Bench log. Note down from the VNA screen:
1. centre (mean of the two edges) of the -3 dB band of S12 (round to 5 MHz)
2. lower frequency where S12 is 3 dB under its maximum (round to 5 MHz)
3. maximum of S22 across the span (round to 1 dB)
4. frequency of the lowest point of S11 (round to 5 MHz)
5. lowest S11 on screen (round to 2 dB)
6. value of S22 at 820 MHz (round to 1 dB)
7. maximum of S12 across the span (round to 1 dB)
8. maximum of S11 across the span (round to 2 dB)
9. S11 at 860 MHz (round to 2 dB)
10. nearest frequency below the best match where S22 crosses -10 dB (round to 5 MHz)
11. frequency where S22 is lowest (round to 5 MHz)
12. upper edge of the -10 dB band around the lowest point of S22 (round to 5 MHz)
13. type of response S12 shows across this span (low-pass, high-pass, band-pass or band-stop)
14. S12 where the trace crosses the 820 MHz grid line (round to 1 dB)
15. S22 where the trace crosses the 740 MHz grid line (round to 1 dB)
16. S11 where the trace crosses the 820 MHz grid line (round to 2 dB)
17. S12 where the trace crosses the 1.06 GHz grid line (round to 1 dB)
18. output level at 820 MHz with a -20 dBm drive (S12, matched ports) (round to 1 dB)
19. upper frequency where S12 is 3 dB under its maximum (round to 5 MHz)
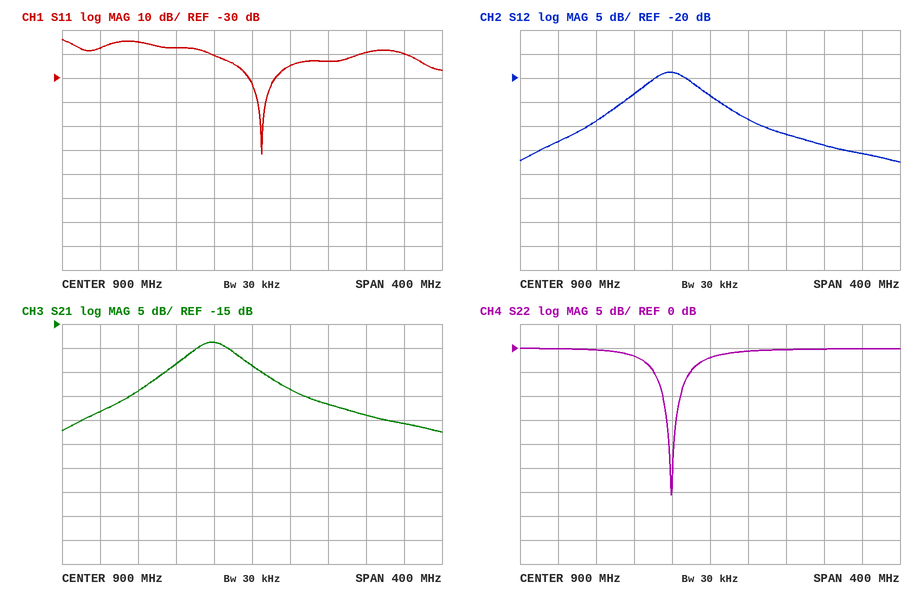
860 MHz
830 MHz
0 dB
910 MHz
-62 dB
-2 dB
-19 dB
-14 dB
-20 dB
850 MHz
860 MHz
870 MHz
band-pass
-23 dB
0 dB
-18 dB
-36 dB
-43 dBm
885 MHz
